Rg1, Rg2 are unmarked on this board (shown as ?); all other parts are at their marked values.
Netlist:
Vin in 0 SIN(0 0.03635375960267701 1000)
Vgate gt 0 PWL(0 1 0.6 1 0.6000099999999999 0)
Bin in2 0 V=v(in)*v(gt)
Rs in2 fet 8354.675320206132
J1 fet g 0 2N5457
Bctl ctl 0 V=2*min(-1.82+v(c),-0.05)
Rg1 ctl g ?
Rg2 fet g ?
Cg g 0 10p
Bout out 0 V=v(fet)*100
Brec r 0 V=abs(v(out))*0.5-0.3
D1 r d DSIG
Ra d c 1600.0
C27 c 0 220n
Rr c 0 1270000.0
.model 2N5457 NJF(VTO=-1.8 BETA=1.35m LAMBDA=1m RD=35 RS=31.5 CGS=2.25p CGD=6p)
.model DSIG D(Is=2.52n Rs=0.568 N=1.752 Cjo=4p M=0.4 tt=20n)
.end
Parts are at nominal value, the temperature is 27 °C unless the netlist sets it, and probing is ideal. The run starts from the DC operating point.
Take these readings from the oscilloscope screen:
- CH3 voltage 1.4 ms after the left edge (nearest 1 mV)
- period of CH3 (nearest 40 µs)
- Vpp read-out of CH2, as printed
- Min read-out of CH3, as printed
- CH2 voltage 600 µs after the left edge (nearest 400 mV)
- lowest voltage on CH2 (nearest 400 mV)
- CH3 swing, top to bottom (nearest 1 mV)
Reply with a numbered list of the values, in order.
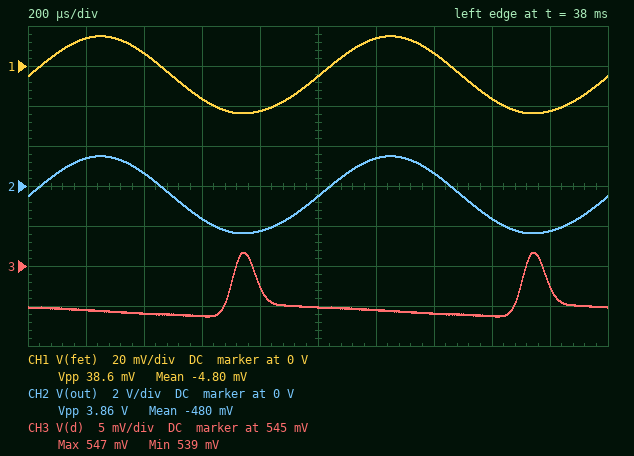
1. 539 mV
2. 1.00 ms
3. 3.86 V
4. 539 mV
5. -1.6 V
6. -2.4 V
7. 8 mV
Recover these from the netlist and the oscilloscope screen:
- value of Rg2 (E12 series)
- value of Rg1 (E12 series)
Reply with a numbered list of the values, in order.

1. 1.5 MΩ
2. 680 kΩ
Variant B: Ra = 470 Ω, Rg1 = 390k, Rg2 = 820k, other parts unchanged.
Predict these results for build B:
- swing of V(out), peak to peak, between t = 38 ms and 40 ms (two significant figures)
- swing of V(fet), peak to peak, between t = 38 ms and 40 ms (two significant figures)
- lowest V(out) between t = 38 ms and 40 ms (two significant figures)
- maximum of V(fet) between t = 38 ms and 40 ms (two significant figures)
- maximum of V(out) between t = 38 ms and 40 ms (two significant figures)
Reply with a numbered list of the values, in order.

1. 3.2 V
2. 32 mV
3. -2.3 V
4. 8.5 mV
5. 850 mV
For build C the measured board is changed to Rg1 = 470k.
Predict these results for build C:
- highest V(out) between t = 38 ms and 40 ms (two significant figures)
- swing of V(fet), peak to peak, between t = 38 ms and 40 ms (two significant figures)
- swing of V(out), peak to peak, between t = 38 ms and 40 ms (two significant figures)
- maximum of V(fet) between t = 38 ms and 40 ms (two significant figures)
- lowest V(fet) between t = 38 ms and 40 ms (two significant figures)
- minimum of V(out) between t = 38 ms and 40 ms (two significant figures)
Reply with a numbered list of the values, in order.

1. 1.8 V
2. 44 mV
3. 4.4 V
4. 18 mV
5. -26 mV
6. -2.6 V
